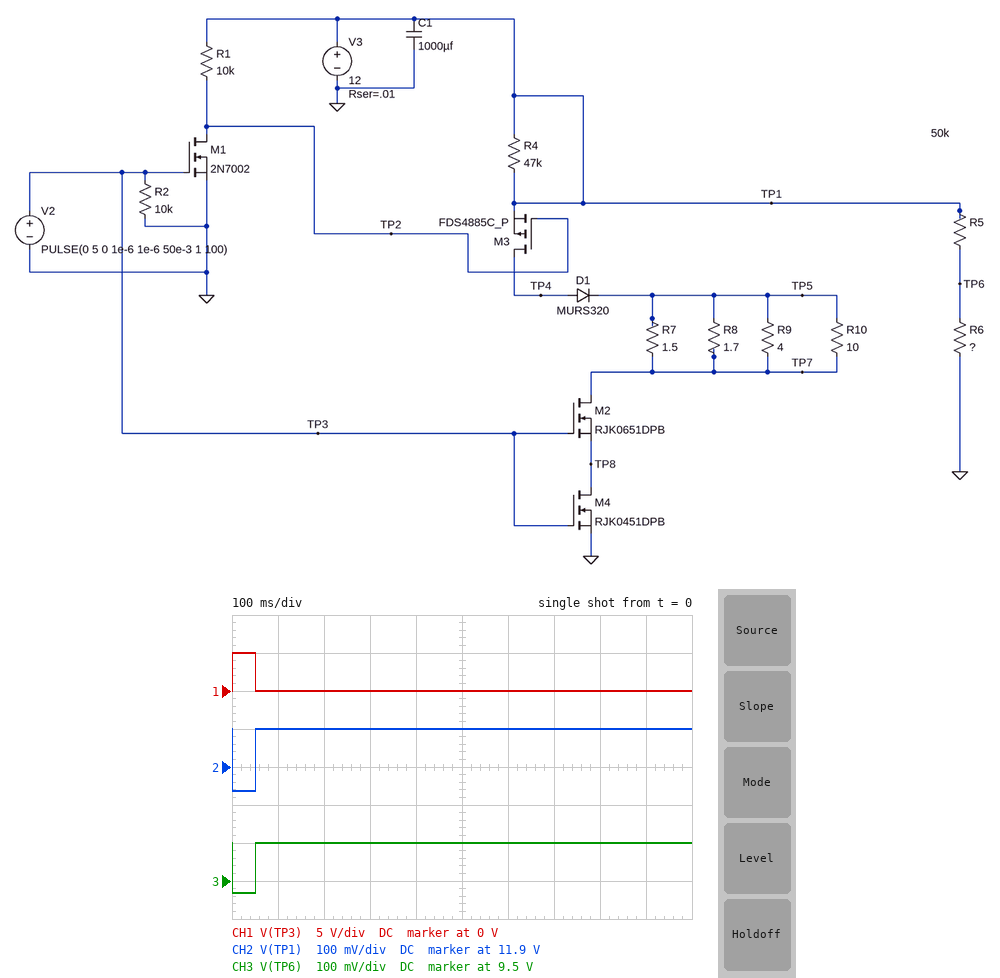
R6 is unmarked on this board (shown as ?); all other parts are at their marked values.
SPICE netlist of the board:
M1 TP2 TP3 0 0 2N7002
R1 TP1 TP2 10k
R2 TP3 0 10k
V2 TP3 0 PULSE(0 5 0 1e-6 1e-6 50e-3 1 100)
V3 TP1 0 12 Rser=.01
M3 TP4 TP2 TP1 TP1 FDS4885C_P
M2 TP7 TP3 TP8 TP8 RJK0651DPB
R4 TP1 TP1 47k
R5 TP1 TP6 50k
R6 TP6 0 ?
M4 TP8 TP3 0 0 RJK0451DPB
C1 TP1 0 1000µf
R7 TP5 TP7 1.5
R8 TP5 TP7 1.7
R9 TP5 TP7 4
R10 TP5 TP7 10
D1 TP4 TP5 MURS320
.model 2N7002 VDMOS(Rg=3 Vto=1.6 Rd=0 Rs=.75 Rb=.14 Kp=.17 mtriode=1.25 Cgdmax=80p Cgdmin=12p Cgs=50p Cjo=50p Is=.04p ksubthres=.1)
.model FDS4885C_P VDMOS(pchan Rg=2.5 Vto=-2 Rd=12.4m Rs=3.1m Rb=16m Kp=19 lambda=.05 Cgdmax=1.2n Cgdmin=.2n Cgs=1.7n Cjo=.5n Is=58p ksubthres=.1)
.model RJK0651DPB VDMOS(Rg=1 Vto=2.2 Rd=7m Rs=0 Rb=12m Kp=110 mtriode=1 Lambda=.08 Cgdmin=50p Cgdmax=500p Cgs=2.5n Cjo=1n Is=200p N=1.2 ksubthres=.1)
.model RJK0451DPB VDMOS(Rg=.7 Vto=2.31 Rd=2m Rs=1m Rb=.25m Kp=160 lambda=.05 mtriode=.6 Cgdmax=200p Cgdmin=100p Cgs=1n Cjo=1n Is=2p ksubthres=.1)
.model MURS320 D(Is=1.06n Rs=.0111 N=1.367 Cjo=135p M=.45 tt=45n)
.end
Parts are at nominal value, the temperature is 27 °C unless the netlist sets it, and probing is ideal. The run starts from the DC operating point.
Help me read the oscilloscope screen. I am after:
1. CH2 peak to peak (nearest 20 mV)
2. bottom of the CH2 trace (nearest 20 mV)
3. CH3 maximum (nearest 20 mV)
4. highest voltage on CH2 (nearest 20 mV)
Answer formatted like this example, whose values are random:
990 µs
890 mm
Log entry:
160 mV
11.84 V
9.60 V
12.00 V
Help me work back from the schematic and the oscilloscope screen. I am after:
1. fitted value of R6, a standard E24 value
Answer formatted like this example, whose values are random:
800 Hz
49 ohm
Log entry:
200 kΩ
